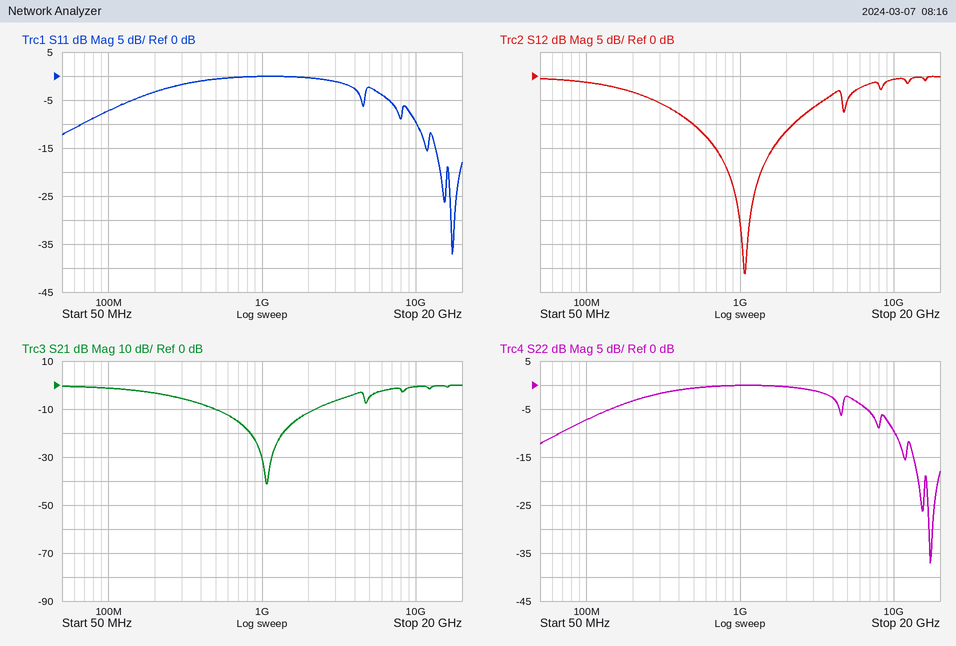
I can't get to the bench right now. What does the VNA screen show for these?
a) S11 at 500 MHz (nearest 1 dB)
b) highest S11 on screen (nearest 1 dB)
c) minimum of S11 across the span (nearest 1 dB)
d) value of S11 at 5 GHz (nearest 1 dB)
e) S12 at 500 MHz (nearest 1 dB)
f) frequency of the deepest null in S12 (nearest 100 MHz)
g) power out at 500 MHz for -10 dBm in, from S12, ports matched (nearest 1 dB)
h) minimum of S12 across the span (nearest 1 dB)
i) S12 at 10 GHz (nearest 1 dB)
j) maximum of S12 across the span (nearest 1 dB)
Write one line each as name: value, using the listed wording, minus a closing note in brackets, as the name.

S11 at 500 MHz: -1 dB
highest S11 on screen: 0 dB
minimum of S11 across the span: -37 dB
value of S11 at 5 GHz: -2 dB
S12 at 500 MHz: -10 dB
frequency of the deepest null in S12: 1.1 GHz
power out at 500 MHz for -10 dBm in, from S12, ports matched: -20 dBm
minimum of S12 across the span: -41 dB
S12 at 10 GHz: -1 dB
maximum of S12 across the span: 0 dB
